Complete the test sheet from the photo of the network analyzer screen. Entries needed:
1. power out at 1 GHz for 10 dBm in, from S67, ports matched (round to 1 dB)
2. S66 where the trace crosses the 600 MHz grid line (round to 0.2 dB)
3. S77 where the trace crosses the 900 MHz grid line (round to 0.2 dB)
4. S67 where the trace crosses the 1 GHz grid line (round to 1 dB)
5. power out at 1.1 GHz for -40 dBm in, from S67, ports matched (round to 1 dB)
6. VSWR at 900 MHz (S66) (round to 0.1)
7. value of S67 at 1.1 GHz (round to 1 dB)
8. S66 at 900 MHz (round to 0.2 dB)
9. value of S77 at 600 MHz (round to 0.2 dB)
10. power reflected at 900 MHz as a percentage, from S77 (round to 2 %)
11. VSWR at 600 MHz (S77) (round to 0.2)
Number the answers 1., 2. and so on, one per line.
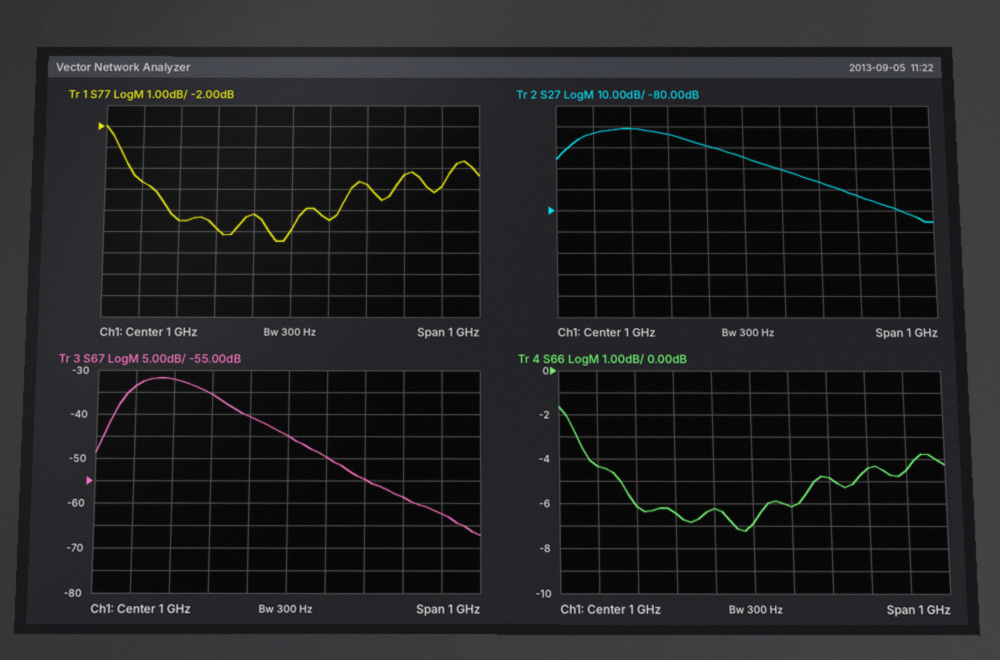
1. -35 dBm
2. -4.4 dB
3. -6.2 dB
4. -45 dB
5. -90 dBm
6. 2.9
7. -50 dB
8. -6.2 dB
9. -4.6 dB
10. 24 %
11. 3.8
